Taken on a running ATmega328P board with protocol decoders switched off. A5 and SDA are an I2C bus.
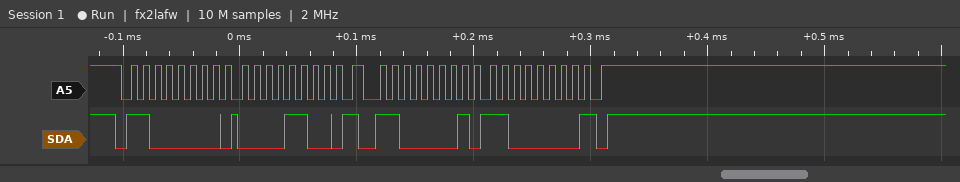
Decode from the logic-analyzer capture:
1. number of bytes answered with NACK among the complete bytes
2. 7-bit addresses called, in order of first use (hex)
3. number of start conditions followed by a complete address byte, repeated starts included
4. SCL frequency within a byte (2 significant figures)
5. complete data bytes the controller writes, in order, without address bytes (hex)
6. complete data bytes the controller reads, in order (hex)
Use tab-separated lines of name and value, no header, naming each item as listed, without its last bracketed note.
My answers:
number of bytes answered with NACK among the complete bytes	1
7-bit addresses called, in order of first use	0x60
number of start conditions followed by a complete address byte, repeated starts included	2
SCL frequency within a byte	100 kHz
complete data bytes the controller writes, in order, without address bytes	0C
complete data bytes the controller reads, in order	C0
